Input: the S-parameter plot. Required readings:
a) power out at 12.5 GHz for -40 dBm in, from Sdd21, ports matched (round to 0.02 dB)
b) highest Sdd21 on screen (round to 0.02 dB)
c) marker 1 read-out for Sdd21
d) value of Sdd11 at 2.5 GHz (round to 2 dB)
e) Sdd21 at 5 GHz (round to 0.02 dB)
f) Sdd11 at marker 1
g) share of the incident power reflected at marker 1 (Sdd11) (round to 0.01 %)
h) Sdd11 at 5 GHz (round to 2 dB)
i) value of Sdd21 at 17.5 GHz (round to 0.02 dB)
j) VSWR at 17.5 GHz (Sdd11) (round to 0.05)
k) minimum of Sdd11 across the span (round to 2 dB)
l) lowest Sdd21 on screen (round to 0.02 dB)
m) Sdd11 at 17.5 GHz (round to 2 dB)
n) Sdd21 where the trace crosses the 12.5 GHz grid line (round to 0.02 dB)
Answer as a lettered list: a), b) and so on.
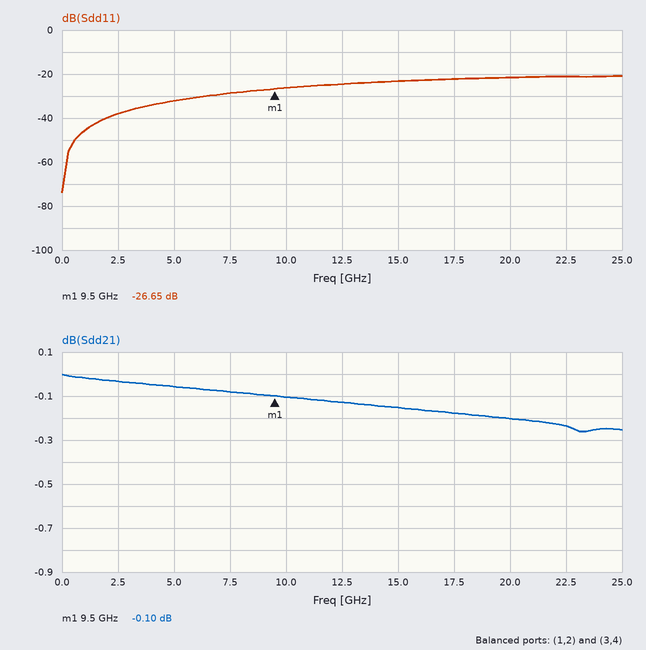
a) -40.12 dBm
b) 0.00 dB
c) -0.10 dB
d) -38 dB
e) -0.06 dB
f) -26.65 dB
g) 0.22 %
h) -32 dB
i) -0.18 dB
j) 1.15
k) -74 dB
l) -0.26 dB
m) -22 dB
n) -0.12 dB
